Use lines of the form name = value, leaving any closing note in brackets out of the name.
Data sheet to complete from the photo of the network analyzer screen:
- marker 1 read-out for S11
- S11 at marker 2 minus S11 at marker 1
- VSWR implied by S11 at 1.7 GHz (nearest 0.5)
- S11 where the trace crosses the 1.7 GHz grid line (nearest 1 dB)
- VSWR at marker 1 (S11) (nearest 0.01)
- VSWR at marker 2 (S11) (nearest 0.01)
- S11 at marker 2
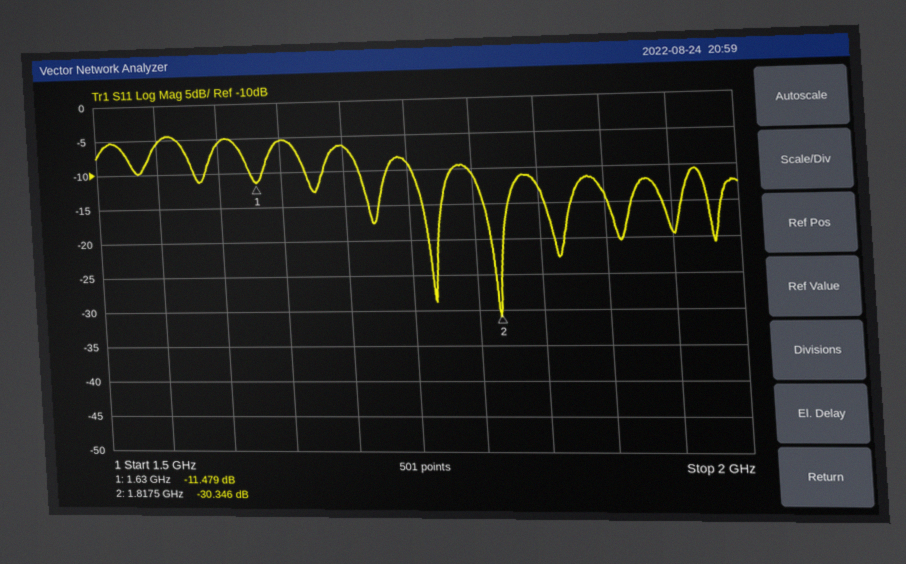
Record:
marker 1 read-out for S11 = -11.479 dB
S11 at marker 2 minus S11 at marker 1 = -18.867 dB
VSWR implied by S11 at 1.7 GHz = 3.0
S11 where the trace crosses the 1.7 GHz grid line = -6 dB
VSWR at marker 1 (S11) = 1.73
VSWR at marker 2 (S11) = 1.06
S11 at marker 2 = -30.346 dB
